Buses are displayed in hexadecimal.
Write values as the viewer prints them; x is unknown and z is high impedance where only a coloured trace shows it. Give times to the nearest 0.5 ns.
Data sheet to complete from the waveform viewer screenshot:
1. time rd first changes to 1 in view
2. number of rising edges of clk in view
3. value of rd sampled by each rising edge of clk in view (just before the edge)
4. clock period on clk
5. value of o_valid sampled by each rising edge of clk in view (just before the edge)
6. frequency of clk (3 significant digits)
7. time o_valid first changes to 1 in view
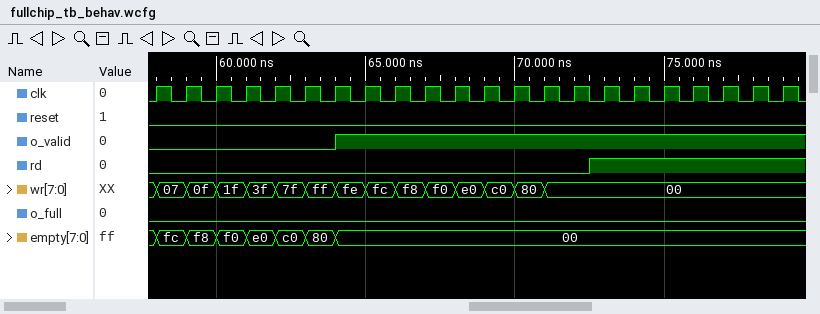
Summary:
72.5 ns
22
0 0 0 0 0 0 0 0 0 0 0 0 0 0 0 1 1 1 1 1 1 1
1 ns
0 0 0 0 0 0 0 1 1 1 1 1 1 1 1 1 1 1 1 1 1 1
1.00 GHz
64 ns
